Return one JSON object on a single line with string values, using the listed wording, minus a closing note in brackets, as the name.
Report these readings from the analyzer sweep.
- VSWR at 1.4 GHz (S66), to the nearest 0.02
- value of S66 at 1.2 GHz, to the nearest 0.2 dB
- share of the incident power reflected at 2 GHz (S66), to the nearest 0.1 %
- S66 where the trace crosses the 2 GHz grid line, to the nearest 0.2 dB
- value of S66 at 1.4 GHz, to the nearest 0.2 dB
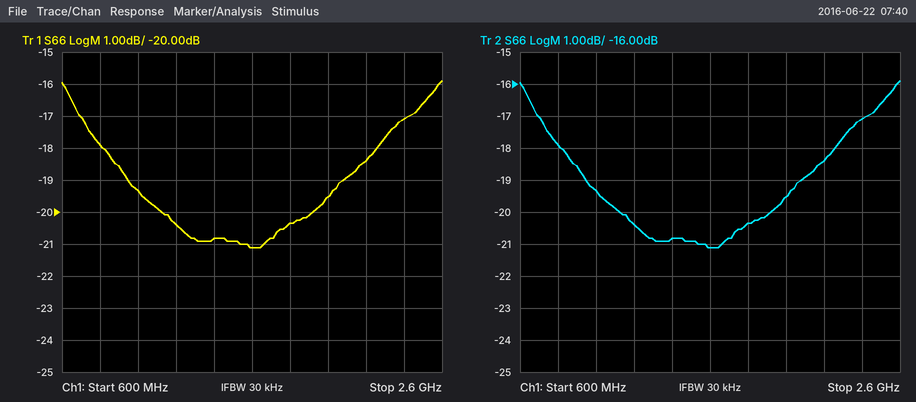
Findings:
{"VSWR at 1.4 GHz (S66), to the nearest 0.02": "1.20", "value of S66 at 1.2 GHz, to the nearest 0.2 dB": "-20.4 dB", "share of the incident power reflected at 2 GHz (S66), to the nearest 0.1 %": "1.1 %", "S66 where the trace crosses the 2 GHz grid line, to the nearest 0.2 dB": "-19.6 dB", "value of S66 at 1.4 GHz, to the nearest 0.2 dB": "-20.8 dB"}
